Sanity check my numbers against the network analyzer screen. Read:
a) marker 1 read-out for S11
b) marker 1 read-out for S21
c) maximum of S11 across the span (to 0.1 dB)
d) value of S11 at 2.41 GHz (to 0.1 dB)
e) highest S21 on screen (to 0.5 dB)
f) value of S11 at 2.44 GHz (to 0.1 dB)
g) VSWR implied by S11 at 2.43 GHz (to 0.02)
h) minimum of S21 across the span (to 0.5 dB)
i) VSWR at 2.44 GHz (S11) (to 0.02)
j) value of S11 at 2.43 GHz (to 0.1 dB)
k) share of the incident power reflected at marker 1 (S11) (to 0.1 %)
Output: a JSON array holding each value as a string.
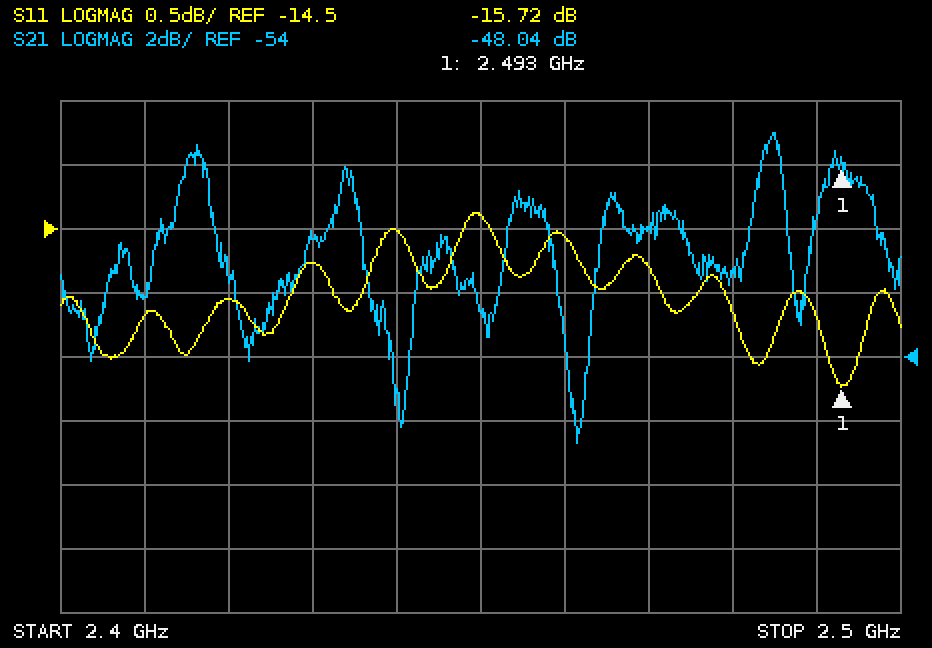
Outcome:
["-15.72 dB", "-48.04 dB", "-14.4 dB", "-15.2 dB", "-47.0 dB", "-14.5 dB", "1.44", "-56.5 dB", "1.46", "-14.8 dB", "2.7 %"]
